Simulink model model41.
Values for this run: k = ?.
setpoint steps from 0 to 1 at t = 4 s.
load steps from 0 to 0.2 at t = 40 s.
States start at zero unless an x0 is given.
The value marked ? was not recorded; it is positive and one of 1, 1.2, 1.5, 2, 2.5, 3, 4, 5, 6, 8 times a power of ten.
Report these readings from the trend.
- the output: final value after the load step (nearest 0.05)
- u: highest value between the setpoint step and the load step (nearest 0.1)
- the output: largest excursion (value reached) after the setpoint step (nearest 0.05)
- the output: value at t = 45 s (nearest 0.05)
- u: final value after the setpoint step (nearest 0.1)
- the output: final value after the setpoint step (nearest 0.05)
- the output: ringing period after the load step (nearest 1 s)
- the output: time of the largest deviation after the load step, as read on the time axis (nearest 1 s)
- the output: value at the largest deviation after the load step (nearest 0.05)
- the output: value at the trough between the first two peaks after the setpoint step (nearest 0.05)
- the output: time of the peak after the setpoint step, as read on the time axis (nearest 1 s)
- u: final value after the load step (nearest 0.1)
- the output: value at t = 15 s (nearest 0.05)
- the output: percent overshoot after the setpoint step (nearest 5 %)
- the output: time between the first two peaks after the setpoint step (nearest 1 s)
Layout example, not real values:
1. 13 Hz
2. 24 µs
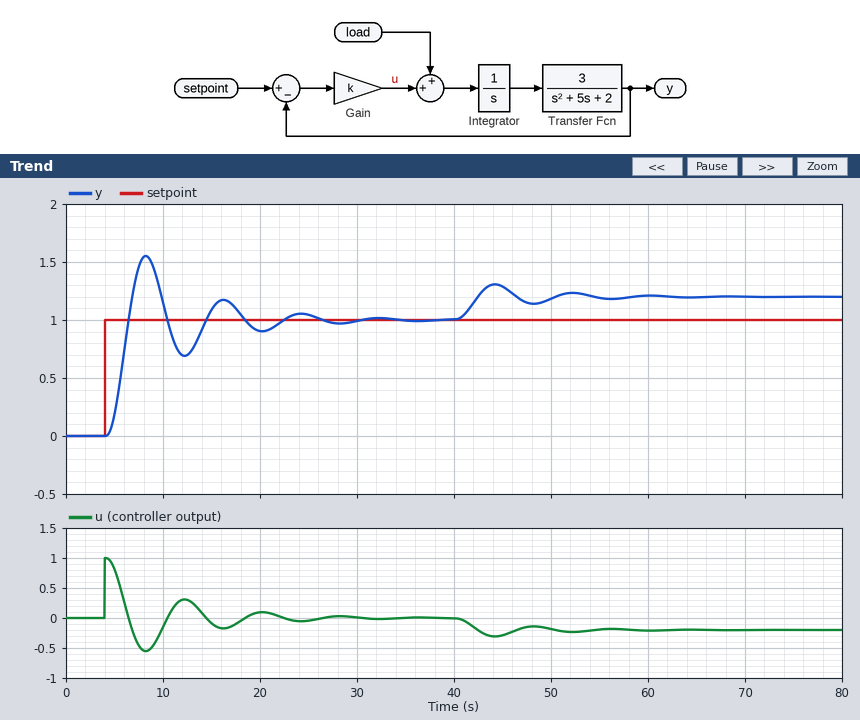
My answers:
1. 1.20
2. 1.0
3. 1.55
4. 1.30
5. 0.0
6. 1.00
7. 8 s
8. 44 s
9. 1.30
10. 0.70
11. 8 s
12. -0.2
13. 1.10
14. 55 %
15. 8 s
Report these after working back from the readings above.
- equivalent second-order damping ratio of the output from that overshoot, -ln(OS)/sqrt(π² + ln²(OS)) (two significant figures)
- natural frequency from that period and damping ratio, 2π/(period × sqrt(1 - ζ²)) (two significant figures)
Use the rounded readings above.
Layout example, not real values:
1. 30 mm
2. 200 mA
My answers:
1. 0.19
2. 0.80 rad/s
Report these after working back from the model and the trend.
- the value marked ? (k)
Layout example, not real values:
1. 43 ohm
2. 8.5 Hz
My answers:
1. 1
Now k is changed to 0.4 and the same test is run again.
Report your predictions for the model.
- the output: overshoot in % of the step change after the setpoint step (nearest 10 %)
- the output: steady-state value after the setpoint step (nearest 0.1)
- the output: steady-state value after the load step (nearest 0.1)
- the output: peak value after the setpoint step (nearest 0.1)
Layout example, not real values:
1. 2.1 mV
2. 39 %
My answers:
1. 30 %
2. 1.0
3. 1.5
4. 1.3
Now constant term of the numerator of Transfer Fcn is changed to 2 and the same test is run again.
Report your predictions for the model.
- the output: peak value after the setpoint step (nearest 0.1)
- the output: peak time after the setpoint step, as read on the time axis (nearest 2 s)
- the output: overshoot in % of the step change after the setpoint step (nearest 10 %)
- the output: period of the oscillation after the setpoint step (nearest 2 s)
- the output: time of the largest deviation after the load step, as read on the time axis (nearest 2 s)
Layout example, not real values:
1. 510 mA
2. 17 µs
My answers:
1. 1.4
2. 10 s
3. 40 %
4. 10 s
5. 46 s
